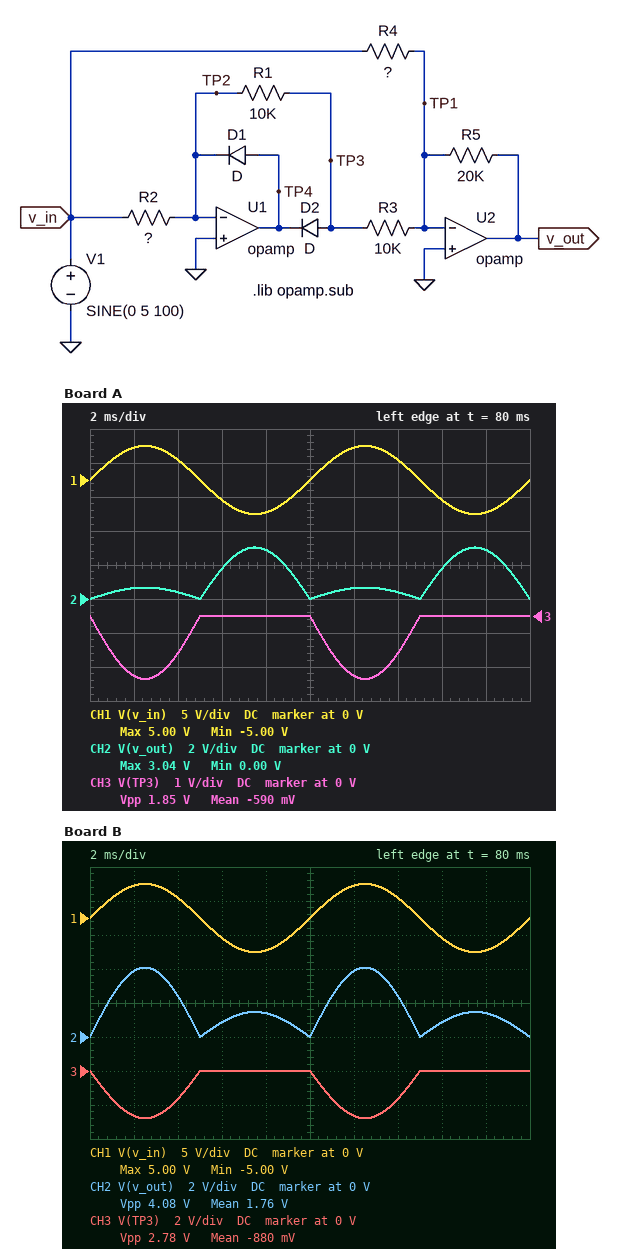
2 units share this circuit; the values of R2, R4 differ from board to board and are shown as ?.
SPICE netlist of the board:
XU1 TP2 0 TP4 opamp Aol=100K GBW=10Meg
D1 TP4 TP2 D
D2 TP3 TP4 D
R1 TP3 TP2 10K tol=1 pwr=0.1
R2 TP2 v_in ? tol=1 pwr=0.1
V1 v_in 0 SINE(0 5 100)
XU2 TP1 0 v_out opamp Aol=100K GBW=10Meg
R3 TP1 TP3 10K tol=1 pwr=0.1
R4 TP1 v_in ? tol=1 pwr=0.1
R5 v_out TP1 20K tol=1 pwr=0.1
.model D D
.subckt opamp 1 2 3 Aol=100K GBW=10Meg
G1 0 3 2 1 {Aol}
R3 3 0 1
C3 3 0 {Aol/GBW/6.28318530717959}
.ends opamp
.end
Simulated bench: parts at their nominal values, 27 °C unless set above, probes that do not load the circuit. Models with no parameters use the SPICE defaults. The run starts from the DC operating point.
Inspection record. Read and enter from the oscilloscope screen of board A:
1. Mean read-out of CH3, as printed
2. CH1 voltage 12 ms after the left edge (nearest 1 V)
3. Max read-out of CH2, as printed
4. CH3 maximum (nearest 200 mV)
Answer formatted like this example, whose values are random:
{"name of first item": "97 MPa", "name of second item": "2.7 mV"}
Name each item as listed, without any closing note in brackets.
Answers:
{"Mean read-out of CH3, as printed": "-590 mV", "CH1 voltage 12 ms after the left edge": "5 V", "Max read-out of CH2, as printed": "3.04 V", "CH3 maximum": "0 V"}
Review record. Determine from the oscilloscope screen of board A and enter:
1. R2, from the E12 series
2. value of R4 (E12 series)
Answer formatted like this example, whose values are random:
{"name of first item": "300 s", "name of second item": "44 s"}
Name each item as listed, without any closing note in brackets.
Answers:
{"R2, from the E12 series": "27 kΩ", "value of R4": "33 kΩ"}
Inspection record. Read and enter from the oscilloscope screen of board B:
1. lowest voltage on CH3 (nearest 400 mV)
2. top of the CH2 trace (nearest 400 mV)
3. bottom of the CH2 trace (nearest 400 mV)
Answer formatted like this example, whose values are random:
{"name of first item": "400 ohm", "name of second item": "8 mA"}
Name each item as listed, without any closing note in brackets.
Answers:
{"lowest voltage on CH3": "-2.8 V", "top of the CH2 trace": "4.0 V", "bottom of the CH2 trace": "0 V"}
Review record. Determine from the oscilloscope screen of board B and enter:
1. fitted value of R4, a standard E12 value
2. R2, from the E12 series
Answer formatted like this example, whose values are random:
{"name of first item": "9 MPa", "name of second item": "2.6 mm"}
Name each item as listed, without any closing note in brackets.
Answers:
{"fitted value of R4, a standard E12 value": "68 kΩ", "R2, from the E12 series": "18 kΩ"}
